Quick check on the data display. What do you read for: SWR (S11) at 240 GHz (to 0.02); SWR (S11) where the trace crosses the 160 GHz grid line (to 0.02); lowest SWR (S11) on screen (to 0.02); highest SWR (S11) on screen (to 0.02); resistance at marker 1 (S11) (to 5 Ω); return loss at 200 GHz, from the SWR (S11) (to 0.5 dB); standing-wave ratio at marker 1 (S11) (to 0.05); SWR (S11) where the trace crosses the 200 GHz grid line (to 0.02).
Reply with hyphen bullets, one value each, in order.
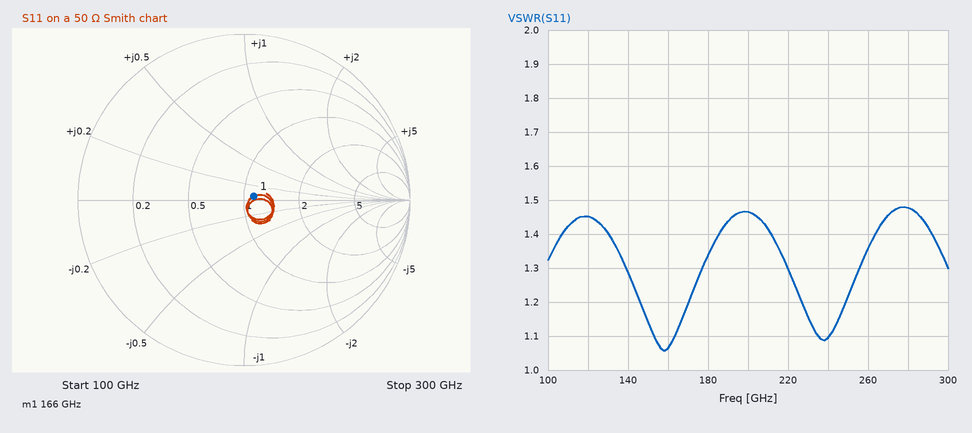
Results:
- 1.10
- 1.06
- 1.06
- 1.48
- 55 Ω
- 14.5 dB
- 1.15
- 1.46
